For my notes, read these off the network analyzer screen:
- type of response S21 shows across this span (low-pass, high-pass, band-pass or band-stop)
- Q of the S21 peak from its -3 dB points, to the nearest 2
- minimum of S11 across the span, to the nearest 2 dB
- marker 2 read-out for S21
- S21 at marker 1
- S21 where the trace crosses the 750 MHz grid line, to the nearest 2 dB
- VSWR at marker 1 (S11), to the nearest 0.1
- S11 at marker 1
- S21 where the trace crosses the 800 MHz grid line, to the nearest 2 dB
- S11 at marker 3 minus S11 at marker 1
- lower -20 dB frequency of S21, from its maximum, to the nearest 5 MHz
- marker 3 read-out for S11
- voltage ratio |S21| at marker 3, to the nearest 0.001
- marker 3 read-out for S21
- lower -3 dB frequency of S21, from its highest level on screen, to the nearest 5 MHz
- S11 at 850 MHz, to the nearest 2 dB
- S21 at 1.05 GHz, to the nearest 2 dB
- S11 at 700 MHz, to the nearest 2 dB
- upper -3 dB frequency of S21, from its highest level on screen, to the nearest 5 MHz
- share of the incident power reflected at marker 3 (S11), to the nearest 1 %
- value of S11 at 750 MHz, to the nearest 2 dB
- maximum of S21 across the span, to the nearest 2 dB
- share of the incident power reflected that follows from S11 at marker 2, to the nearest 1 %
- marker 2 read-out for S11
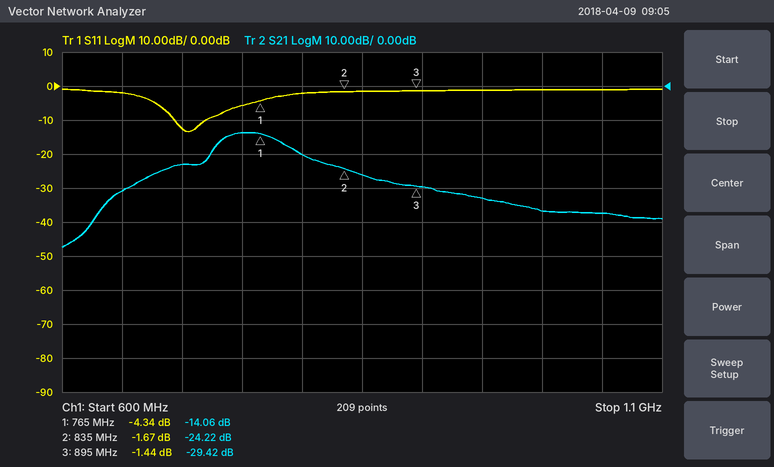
band-pass
14
-14 dB
-24.22 dB
-14.06 dB
-14 dB
4.1
-4.34 dB
-20 dB
2.90 dB
640 MHz
-1.44 dB
0.034
-29.42 dB
730 MHz
-2 dB
-38 dB
-12 dB
785 MHz
72 %
-6 dB
-14 dB
68 %
-1.67 dB
